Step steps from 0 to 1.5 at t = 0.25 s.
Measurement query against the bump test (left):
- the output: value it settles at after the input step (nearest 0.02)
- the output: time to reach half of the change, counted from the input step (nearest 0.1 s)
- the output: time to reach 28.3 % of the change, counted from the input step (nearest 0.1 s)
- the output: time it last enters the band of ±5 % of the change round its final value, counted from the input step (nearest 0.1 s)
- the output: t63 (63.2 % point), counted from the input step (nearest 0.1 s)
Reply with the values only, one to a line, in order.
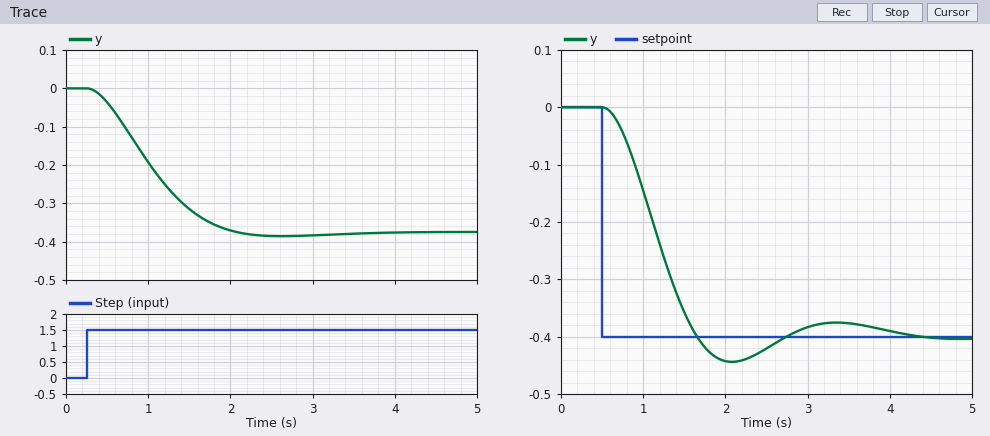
-0.38
0.7 s
0.5 s
1.6 s
0.9 s
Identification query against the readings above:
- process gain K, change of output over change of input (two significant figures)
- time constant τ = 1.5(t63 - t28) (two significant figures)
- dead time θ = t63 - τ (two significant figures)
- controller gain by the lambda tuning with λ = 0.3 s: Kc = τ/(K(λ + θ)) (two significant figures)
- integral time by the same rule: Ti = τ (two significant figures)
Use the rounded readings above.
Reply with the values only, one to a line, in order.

-0.25
0.60 s
0.30 s
-4.0
0.60 s
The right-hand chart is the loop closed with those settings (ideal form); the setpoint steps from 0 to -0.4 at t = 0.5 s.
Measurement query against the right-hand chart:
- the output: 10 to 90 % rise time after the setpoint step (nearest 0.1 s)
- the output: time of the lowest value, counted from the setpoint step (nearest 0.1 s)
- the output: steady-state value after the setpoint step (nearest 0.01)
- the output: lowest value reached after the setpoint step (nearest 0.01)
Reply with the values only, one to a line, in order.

0.8 s
1.6 s
-0.40
-0.44
